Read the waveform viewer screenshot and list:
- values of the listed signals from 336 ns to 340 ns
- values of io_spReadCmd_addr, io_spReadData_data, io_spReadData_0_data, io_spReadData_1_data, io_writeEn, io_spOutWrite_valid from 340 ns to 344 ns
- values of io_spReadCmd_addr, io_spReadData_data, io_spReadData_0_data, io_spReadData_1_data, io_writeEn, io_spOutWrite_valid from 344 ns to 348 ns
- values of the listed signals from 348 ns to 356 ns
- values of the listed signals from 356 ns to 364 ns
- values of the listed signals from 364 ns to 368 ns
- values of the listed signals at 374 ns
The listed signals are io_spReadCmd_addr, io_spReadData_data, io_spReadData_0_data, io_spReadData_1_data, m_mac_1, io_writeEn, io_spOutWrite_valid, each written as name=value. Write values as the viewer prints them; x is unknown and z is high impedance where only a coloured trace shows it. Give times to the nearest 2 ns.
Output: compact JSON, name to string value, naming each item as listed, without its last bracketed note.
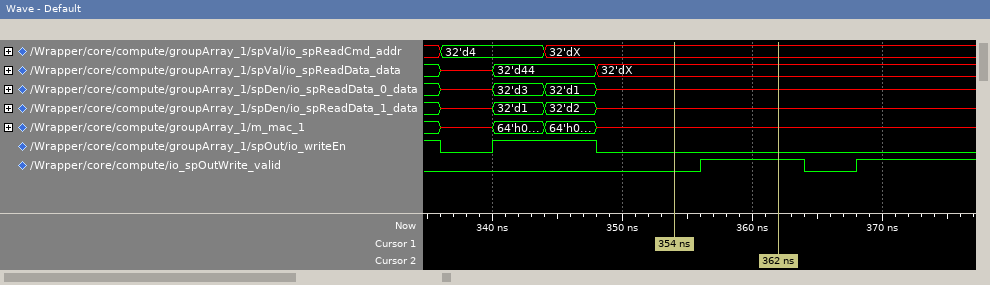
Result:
{"values of the listed signals from 336 ns to 340 ns": "io_spReadCmd_addr=32'd4, io_spReadData_data=x, io_spReadData_0_data=x, io_spReadData_1_data=x, m_mac_1=x, io_writeEn=0, io_spOutWrite_valid=0", "values of io_spReadCmd_addr, io_spReadData_data, io_spReadData_0_data, io_spReadData_1_data, io_writeEn, io_spOutWrite_valid from 340 ns to 344 ns": "io_spReadCmd_addr=32'd4, io_spReadData_data=32'd44, io_spReadData_0_data=32'd3, io_spReadData_1_data=32'd1, io_writeEn=1, io_spOutWrite_valid=0", "values of io_spReadCmd_addr, io_spReadData_data, io_spReadData_0_data, io_spReadData_1_data, io_writeEn, io_spOutWrite_valid from 344 ns to 348 ns": "io_spReadCmd_addr=32'dX, io_spReadData_data=32'd44, io_spReadData_0_data=32'd1, io_spReadData_1_data=32'd2, io_writeEn=1, io_spOutWrite_valid=0", "values of the listed signals from 348 ns to 356 ns": "io_spReadCmd_addr=32'dX, io_spReadData_data=32'dX, io_spReadData_0_data=x, io_spReadData_1_data=x, m_mac_1=x, io_writeEn=0, io_spOutWrite_valid=0", "values of the listed signals from 356 ns to 364 ns": "io_spReadCmd_addr=32'dX, io_spReadData_data=32'dX, io_spReadData_0_data=x, io_spReadData_1_data=x, m_mac_1=x, io_writeEn=0, io_spOutWrite_valid=1", "values of the listed signals from 364 ns to 368 ns": "io_spReadCmd_addr=32'dX, io_spReadData_data=32'dX, io_spReadData_0_data=x, io_spReadData_1_data=x, m_mac_1=x, io_writeEn=0, io_spOutWrite_valid=0", "values of the listed signals at 374 ns": "io_spReadCmd_addr=32'dX, io_spReadData_data=32'dX, io_spReadData_0_data=x, io_spReadData_1_data=x, m_mac_1=x, io_writeEn=0, io_spOutWrite_valid=1"}
